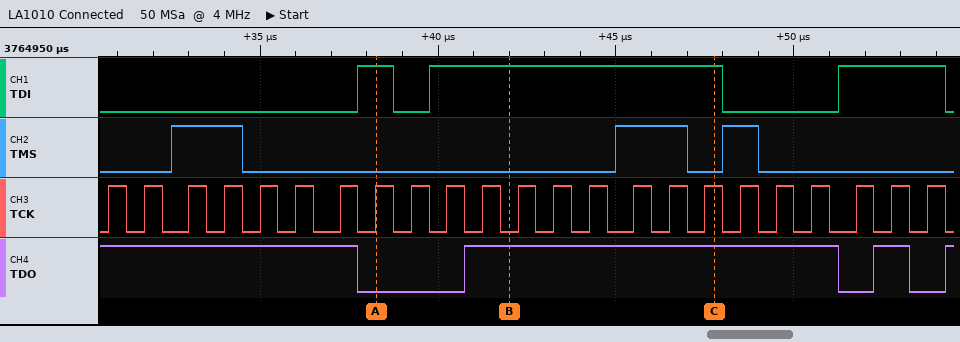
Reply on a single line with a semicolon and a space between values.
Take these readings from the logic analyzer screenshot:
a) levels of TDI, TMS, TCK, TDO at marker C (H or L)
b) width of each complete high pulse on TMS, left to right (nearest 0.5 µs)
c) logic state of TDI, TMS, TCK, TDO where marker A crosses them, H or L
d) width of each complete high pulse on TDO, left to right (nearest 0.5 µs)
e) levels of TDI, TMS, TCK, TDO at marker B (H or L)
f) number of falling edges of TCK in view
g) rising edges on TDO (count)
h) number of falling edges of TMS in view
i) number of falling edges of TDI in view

TDI=H, TMS=L, TCK=H, TDO=H; 2 µs, 2 µs, 1 µs; TDI=H, TMS=L, TCK=H, TDO=L; 10.5 µs, 1 µs; TDI=H, TMS=L, TCK=L, TDO=H; 23; 3; 3; 3
